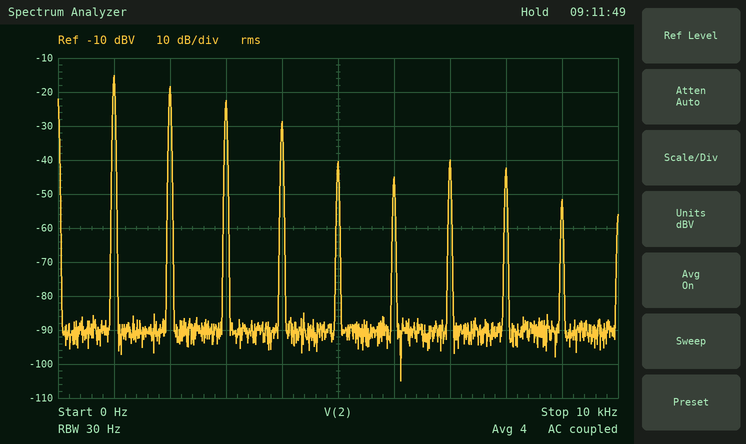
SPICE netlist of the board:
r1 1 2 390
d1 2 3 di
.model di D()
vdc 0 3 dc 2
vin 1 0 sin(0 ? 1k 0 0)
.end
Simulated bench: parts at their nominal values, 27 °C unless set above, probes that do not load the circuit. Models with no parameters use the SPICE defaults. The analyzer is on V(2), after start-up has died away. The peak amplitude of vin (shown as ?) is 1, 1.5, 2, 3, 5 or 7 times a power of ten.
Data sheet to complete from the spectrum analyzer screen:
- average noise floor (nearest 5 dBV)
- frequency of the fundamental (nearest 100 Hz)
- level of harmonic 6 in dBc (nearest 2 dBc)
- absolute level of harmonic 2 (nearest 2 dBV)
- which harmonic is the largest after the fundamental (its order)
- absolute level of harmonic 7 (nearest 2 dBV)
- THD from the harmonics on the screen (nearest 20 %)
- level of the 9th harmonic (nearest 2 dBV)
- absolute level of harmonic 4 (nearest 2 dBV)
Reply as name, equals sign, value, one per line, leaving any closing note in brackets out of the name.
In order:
average noise floor = -90 dBV
frequency of the fundamental = 1.0 kHz
level of harmonic 6 in dBc = -30 dBc
absolute level of harmonic 2 = -18 dBV
which harmonic is the largest after the fundamental = 2
absolute level of harmonic 7 = -40 dBV
THD from the harmonics on the screen = 80 %
level of the 9th harmonic = -52 dBV
absolute level of harmonic 4 = -28 dBV
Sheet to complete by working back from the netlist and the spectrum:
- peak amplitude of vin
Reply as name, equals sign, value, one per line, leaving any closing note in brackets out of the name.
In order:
peak amplitude of vin = 2 V
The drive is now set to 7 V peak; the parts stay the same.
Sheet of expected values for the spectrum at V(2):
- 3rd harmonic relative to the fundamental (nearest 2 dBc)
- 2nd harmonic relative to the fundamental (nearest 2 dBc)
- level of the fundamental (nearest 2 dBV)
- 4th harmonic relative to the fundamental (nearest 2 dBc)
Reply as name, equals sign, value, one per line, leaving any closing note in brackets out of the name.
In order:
3rd harmonic relative to the fundamental = -20 dBc
2nd harmonic relative to the fundamental = -6 dBc
level of the fundamental = 6 dBV
4th harmonic relative to the fundamental = -22 dBc
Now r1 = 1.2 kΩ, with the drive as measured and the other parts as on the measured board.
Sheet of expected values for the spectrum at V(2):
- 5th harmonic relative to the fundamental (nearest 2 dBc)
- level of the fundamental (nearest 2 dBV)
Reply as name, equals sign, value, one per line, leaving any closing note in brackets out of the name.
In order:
5th harmonic relative to the fundamental = -24 dBc
level of the fundamental = -16 dBV
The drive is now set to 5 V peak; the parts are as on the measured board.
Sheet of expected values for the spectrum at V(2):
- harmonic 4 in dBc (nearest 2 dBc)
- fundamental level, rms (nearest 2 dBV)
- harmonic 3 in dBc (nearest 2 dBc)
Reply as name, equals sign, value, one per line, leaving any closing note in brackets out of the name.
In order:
harmonic 4 in dBc = -24 dBc
fundamental level, rms = 2 dBV
harmonic 3 in dBc = -16 dBc
